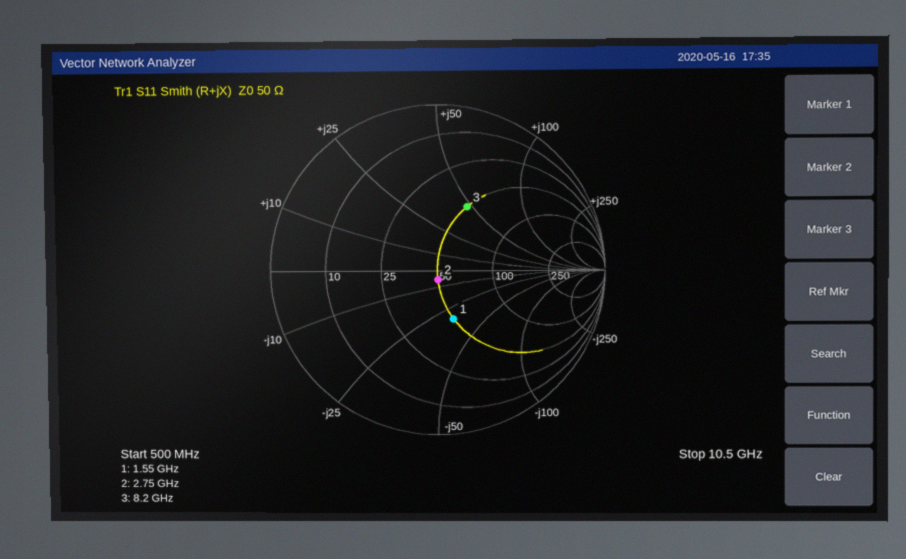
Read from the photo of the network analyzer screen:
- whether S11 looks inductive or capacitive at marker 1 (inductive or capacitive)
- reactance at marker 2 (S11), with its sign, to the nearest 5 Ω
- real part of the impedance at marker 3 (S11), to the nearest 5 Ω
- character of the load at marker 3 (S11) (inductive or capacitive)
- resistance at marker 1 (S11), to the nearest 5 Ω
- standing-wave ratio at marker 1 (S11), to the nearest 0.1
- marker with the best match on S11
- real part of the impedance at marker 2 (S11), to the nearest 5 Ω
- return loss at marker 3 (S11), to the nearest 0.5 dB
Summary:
capacitive
-5 Ω
50 Ω
inductive
50 Ω
1.9
marker 2
50 Ω
7.5 dB
